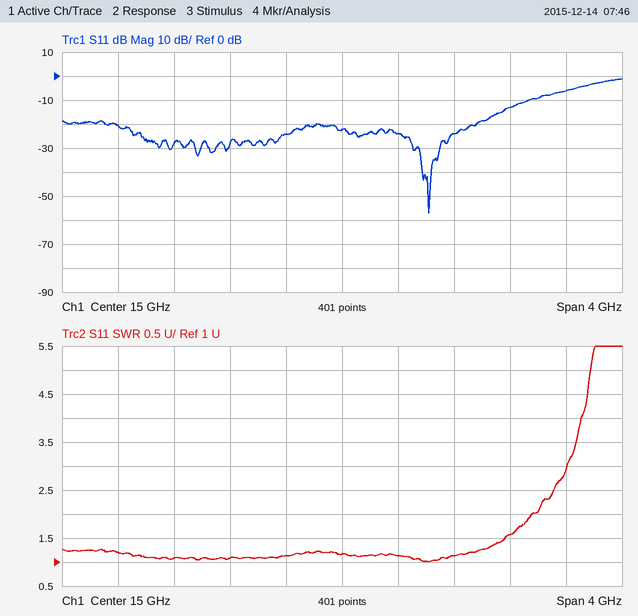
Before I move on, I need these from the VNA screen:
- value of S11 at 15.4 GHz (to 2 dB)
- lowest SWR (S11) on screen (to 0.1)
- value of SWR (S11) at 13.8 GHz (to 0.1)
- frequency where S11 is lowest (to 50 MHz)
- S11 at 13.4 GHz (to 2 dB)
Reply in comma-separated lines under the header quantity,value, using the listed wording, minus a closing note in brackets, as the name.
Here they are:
quantity,value
value of S11 at 15.4 GHz,-24 dB
lowest SWR (S11) on screen,1.0
value of SWR (S11) at 13.8 GHz,1.1
frequency where S11 is lowest,15.60 GHz
S11 at 13.4 GHz,-20 dB
